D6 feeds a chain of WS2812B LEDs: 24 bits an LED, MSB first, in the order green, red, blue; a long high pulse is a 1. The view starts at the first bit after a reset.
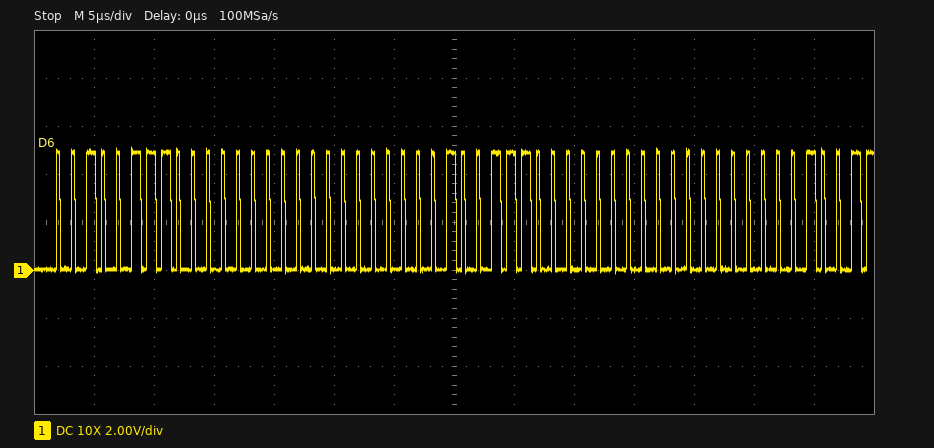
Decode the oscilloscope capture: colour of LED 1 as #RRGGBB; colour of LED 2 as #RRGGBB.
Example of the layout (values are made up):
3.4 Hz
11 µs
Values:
#002700
#002700
